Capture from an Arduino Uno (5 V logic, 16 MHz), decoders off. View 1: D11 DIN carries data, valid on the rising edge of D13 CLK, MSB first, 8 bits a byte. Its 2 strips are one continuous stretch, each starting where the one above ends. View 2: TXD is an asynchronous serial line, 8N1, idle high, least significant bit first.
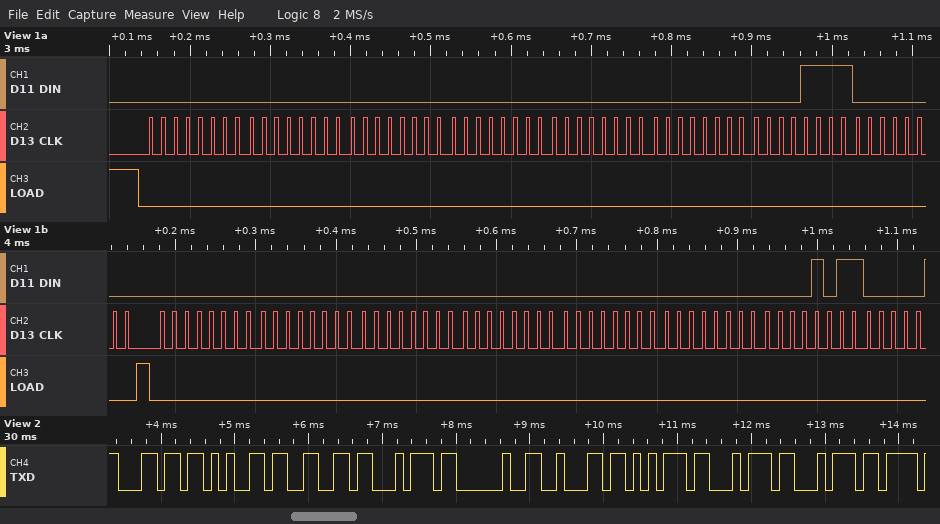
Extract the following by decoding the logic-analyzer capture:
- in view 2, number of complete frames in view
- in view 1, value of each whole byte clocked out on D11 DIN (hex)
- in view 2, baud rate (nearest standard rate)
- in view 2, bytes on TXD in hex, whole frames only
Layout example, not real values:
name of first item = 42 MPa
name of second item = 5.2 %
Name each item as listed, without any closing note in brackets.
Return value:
in view 2, number of complete frames in view = 9
in view 1, value of each whole byte clocked out on D11 DIN = 00 00 00 00 00 00 0F 00 00 00 00 00 00 00 0B
in view 2, baud rate = 9600 baud
in view 2, bytes on TXD in hex, whole frames only = 6C 65 66 74 20 62 75 74 74
